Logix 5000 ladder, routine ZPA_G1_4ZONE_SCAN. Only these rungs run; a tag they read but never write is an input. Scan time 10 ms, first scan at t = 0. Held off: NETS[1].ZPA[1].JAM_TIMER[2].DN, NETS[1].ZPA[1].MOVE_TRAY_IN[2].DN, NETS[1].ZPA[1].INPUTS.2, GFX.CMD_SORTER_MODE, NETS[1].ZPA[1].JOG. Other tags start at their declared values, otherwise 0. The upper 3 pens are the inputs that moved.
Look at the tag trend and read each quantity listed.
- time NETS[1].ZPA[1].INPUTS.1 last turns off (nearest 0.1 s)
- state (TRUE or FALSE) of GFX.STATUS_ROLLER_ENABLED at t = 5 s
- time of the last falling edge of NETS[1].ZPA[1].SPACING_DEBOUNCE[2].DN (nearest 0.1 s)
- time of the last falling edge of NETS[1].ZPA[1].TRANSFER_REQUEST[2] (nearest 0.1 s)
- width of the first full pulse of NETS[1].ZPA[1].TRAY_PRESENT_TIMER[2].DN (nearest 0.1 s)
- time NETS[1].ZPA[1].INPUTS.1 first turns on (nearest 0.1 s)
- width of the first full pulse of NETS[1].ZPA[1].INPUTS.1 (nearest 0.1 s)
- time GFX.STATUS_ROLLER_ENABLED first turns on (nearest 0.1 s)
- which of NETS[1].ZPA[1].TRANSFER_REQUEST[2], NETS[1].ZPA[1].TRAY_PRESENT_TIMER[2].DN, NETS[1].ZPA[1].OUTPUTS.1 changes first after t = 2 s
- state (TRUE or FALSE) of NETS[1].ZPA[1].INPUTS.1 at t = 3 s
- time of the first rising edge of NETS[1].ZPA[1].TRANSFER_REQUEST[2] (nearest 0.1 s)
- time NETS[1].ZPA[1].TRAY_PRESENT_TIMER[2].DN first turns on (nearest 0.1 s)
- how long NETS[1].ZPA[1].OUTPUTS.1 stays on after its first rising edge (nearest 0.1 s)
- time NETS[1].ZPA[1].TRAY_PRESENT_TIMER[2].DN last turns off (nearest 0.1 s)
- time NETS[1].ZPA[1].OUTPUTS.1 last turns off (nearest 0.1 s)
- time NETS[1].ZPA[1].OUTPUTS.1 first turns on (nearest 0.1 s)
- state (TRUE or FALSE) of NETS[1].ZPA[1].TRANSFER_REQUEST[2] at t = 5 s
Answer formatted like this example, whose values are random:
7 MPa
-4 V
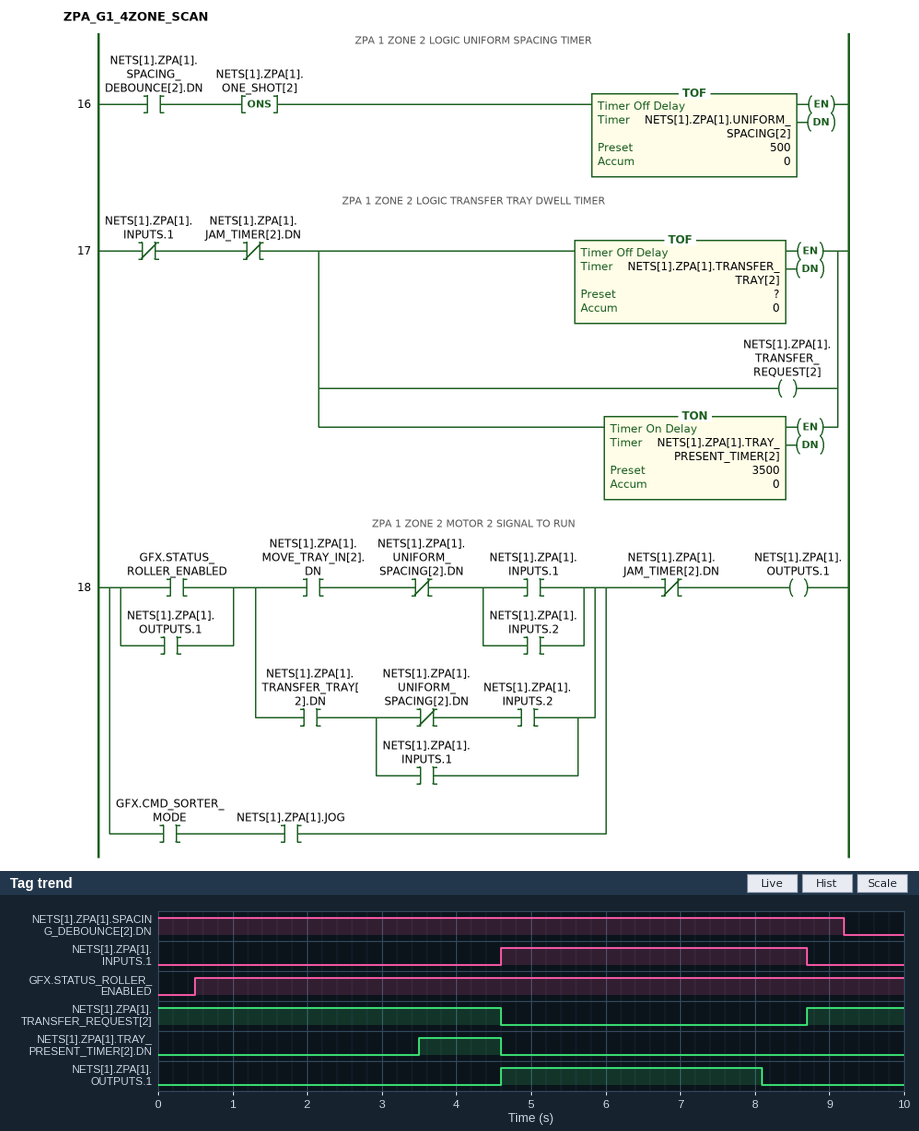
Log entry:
8.7 s
TRUE
9.2 s
4.6 s
1.1 s
4.6 s
4.1 s
0.5 s
NETS[1].ZPA[1].TRAY_PRESENT_TIMER[2].DN
FALSE
8.7 s
3.5 s
3.5 s
4.6 s
8.1 s
4.6 s
FALSE
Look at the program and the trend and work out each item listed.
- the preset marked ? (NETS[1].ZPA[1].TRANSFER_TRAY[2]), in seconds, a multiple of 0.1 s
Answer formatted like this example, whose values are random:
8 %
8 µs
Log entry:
3.5 s
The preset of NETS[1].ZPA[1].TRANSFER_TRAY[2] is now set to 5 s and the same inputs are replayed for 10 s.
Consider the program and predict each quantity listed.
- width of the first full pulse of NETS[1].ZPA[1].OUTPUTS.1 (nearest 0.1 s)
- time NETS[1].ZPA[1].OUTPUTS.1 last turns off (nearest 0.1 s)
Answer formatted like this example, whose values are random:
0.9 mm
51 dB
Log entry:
4.1 s
8.7 s
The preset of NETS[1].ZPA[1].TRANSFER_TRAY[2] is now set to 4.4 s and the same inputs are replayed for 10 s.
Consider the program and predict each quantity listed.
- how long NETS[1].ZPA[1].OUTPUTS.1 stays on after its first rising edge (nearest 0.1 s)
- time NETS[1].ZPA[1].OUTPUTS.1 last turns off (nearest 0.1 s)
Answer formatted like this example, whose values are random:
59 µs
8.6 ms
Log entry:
4.1 s
8.7 s
